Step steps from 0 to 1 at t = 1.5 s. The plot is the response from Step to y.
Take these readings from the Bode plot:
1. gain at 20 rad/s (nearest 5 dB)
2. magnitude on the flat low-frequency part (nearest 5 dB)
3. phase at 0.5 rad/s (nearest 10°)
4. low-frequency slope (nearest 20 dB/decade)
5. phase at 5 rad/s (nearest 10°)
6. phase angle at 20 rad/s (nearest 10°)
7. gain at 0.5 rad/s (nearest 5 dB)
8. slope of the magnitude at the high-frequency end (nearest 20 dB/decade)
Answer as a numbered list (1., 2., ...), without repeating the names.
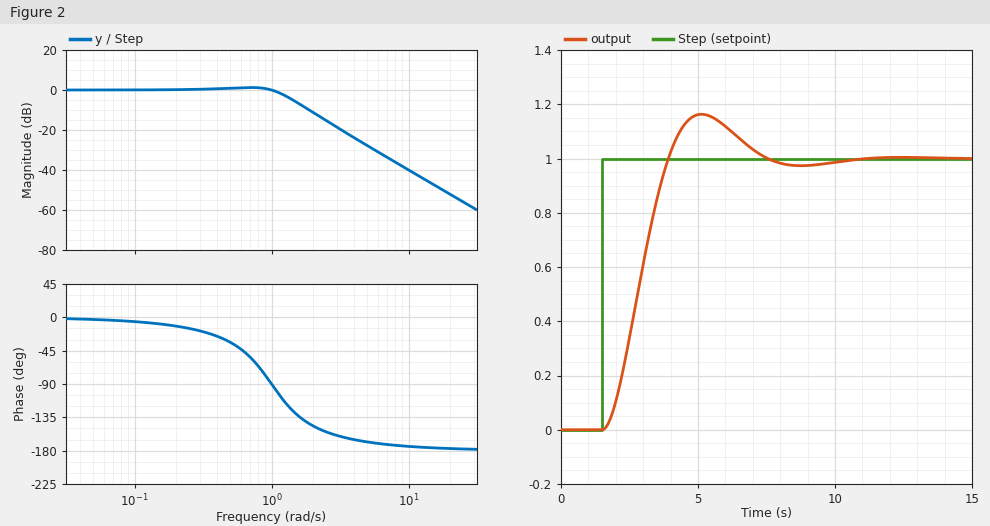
1. -50 dB
2. 0 dB
3. -30°
4. 0 dB/decade
5. -170°
6. -180°
7. 0 dB
8. -40 dB/decade
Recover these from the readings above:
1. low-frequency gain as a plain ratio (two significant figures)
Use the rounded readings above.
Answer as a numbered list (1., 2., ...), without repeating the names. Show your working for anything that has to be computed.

1. 10^(0 / 20) = 1.0
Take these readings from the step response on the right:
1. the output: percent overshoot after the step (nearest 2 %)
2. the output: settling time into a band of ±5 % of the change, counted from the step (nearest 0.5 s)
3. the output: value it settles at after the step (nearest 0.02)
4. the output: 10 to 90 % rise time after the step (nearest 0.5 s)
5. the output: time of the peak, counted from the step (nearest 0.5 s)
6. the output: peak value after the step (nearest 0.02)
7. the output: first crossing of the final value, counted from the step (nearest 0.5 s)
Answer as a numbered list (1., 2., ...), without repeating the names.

1. 16 %
2. 5.5 s
3. 1.00
4. 1.5 s
5. 3.5 s
6. 1.16
7. 2.5 s
